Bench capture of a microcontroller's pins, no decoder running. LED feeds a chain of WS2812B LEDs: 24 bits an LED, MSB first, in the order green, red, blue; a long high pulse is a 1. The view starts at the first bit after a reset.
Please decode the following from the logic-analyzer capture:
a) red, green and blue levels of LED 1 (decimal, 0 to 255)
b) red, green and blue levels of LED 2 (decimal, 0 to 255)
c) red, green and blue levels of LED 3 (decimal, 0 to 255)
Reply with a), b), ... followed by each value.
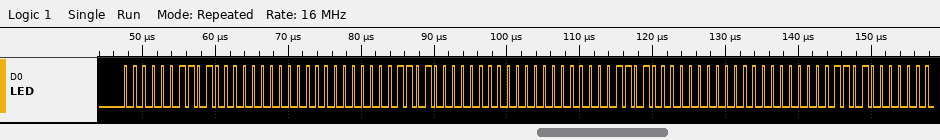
a) 64, 3, 0
b) 64, 3, 0
c) 64, 3, 0
